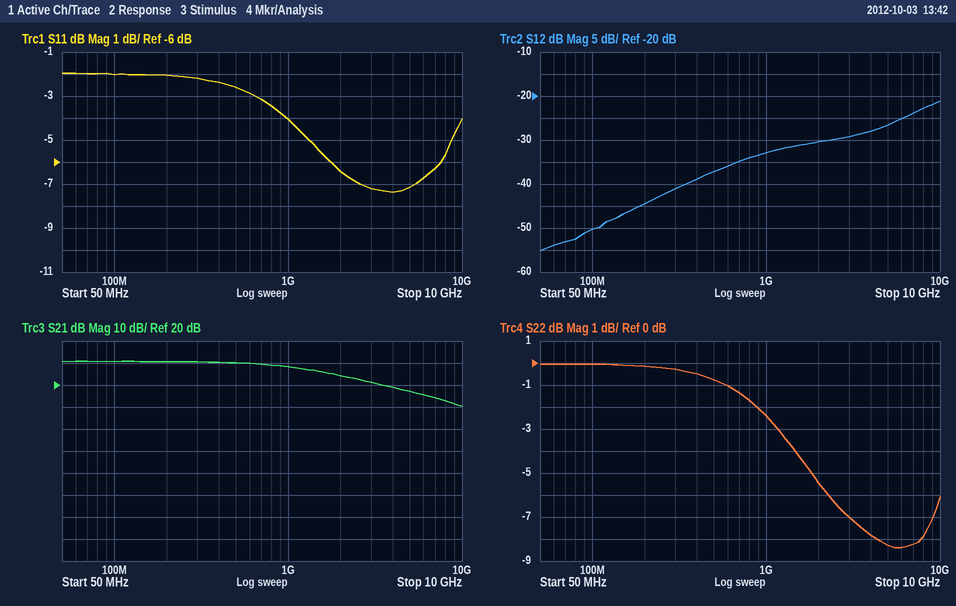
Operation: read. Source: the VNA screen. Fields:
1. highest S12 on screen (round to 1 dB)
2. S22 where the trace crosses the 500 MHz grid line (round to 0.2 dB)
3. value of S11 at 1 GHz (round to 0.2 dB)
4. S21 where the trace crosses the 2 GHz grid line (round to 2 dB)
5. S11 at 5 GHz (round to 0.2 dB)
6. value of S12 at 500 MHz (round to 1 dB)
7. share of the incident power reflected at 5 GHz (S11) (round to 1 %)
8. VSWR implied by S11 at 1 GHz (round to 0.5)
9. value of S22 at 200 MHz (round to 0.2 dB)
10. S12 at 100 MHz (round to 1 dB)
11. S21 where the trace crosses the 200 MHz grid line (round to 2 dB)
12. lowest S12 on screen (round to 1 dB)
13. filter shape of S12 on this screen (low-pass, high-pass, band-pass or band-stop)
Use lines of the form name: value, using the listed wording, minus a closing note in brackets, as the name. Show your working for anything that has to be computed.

highest S12 on screen: -21 dB
S22 where the trace crosses the 500 MHz grid line: -0.8 dB
value of S11 at 1 GHz: -4.0 dB
S21 where the trace crosses the 2 GHz grid line: 24 dB
S11 at 5 GHz: -7.2 dB
value of S12 at 500 MHz: -37 dB
share of the incident power reflected at 5 GHz (S11): 10^(-7.2/10) ≈ 19 %
VSWR implied by S11 at 1 GHz: |Γ| = 10^(-4/20) = 0.6310; VSWR = (1 + 0.6310)/(1 − 0.6310) ≈ 4.42, so 4.5 to the nearest 0.5
value of S22 at 200 MHz: -0.2 dB
S12 at 100 MHz: -50 dB
S21 where the trace crosses the 200 MHz grid line: 30 dB
lowest S12 on screen: -55 dB
filter shape of S12 on this screen: high-pass
